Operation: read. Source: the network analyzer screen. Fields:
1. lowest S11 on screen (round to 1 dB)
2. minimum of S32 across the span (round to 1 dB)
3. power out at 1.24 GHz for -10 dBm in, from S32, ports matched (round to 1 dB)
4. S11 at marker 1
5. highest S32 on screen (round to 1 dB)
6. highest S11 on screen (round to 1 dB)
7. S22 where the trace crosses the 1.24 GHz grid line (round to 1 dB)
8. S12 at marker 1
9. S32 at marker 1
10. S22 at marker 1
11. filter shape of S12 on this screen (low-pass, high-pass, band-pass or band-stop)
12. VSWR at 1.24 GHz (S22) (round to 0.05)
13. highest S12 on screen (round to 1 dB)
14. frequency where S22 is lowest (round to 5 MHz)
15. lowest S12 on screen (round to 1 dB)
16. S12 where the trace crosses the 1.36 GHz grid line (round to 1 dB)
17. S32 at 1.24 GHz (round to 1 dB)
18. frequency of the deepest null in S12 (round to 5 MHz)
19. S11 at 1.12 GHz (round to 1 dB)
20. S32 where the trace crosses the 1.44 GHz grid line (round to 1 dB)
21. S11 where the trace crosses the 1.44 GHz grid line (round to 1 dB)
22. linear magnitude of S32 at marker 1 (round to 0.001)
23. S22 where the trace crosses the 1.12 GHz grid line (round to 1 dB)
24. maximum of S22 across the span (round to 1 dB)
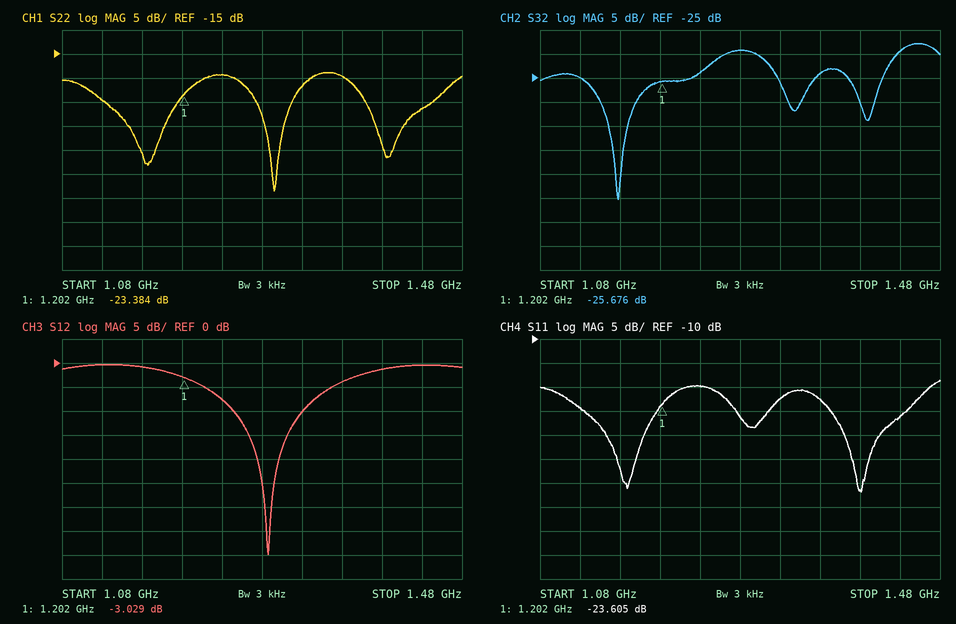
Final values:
-42 dB
-50 dB
-34 dBm
-23.605 dB
-18 dB
-19 dB
-19 dB
-3.029 dB
-25.676 dB
-23.384 dB
band-stop
1.25
0 dB
1.290 GHz
-40 dB
-4 dB
-24 dB
1.285 GHz
-24 dB
-19 dB
-26 dB
0.052
-25 dB
-19 dB
